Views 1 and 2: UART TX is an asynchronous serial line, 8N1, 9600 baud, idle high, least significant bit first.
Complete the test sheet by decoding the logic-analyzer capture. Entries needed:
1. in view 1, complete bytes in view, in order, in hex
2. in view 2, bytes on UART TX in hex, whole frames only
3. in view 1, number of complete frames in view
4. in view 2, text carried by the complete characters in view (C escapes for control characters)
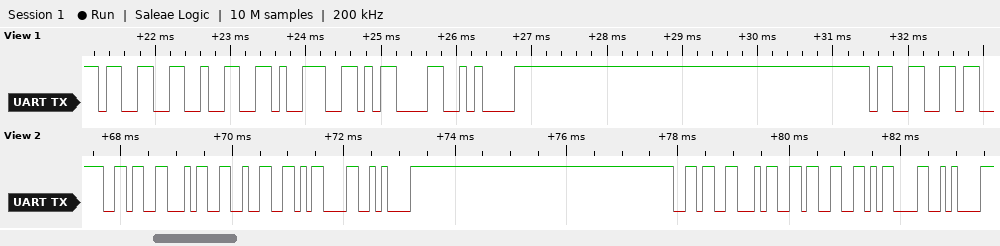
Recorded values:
33 32 39 0D 0A 33
36 34 32 0D 0A 36 34 33 0D 0A
6
"642\r\n643\r\n"
